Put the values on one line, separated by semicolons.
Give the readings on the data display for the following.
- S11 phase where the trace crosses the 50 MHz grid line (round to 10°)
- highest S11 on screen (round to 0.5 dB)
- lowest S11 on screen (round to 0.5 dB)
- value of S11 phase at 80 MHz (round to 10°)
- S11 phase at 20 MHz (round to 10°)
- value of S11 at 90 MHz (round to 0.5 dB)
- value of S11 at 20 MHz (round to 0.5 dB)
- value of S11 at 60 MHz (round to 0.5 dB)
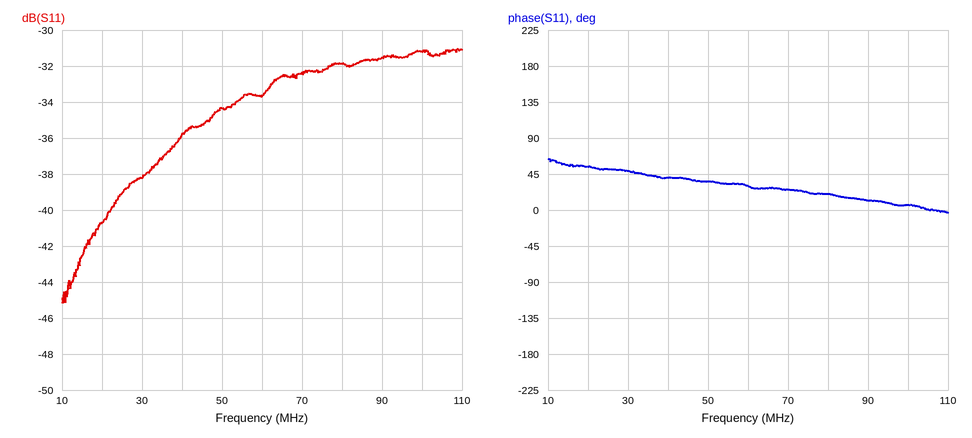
40°; -31.0 dB; -45.0 dB; 20°; 50°; -31.5 dB; -40.5 dB; -33.5 dB
